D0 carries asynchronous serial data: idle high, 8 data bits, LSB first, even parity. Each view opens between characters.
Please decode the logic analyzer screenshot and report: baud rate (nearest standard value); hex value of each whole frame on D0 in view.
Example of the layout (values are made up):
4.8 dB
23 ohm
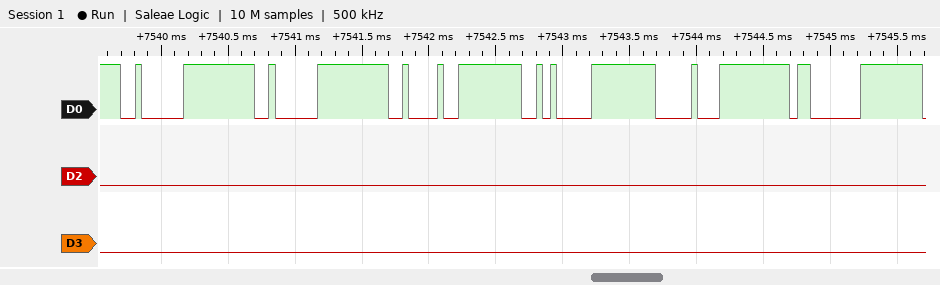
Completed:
19200 baud
02, 02, 42, 0A, 10, 03
